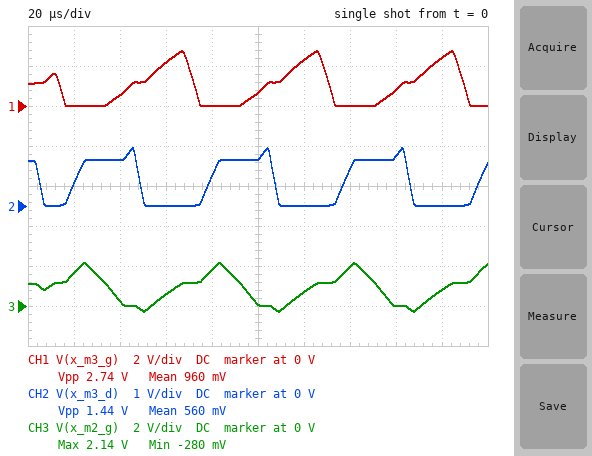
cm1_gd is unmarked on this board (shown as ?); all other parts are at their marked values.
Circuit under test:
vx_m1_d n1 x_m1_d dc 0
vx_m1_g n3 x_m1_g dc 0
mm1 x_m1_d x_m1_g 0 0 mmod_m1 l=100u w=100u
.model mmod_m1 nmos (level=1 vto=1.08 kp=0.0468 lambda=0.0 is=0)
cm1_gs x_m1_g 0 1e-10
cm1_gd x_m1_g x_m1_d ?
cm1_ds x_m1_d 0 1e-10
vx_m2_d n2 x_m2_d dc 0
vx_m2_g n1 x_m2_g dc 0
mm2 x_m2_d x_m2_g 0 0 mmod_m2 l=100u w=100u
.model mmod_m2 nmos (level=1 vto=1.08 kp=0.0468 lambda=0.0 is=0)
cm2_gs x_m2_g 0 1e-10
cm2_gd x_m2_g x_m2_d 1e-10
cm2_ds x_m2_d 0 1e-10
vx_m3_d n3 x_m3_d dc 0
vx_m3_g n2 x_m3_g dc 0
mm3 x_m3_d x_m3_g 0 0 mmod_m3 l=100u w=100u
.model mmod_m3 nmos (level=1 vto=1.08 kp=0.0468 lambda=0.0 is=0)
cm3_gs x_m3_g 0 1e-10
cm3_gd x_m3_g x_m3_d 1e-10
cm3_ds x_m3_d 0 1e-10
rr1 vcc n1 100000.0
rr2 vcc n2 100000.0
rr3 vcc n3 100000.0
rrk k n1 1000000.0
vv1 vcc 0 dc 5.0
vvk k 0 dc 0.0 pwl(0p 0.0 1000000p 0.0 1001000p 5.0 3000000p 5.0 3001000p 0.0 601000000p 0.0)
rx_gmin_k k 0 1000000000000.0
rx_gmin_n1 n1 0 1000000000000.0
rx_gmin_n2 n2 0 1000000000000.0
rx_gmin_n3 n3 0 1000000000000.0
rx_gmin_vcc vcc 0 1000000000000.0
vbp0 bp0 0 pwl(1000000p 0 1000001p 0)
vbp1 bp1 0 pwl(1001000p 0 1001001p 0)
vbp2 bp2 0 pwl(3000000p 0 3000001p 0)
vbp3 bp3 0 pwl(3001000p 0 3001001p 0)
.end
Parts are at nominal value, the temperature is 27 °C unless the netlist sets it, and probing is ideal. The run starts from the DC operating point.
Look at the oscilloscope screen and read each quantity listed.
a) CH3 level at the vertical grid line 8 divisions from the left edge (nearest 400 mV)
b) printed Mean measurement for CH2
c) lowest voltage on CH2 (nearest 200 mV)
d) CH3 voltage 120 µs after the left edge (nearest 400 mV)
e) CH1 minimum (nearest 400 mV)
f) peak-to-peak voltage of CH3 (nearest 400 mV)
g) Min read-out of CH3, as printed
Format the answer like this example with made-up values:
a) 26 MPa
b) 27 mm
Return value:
a) 0 V
b) 560 mV
c) 0 V
d) 800 mV
e) 0 V
f) 2.4 V
g) -280 mV
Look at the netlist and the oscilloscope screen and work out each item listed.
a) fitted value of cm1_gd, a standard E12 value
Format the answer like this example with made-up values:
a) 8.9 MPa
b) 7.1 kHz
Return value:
a) 330 pF
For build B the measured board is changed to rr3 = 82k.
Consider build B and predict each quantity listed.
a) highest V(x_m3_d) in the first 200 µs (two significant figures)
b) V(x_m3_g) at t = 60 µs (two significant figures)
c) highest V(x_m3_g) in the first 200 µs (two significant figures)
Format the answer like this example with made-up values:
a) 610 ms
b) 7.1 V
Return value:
a) 1.6 V
b) 2.5 V
c) 2.7 V
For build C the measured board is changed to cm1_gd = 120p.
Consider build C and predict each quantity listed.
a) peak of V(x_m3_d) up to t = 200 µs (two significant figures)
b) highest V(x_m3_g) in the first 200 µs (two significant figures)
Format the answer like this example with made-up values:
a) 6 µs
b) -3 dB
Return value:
a) 2.0 V
b) 2.1 V
